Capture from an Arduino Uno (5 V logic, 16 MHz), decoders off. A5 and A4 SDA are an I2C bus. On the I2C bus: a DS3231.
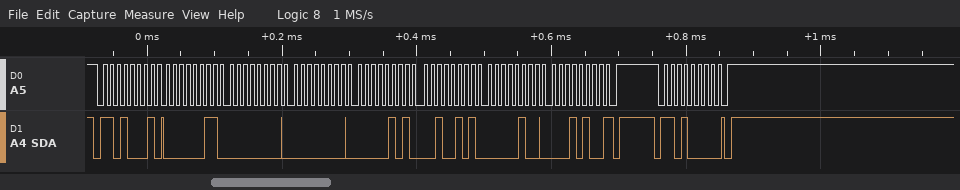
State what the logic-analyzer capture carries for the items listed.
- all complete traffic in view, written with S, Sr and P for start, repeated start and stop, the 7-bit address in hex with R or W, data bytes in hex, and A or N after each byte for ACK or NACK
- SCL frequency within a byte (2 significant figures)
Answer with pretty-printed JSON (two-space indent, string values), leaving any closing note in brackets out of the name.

{
  "all complete traffic in view, written with S, Sr and P for start, repeated start and stop, the 7-bit address in hex with R or W, data bytes in hex, and A or N after each byte for ACK or NACK": "S 68R A 03 A 00 A 00 A 05 A 25 A 04 A 14 N P S 68W A P",
  "SCL frequency within a byte": "100 kHz"
}
